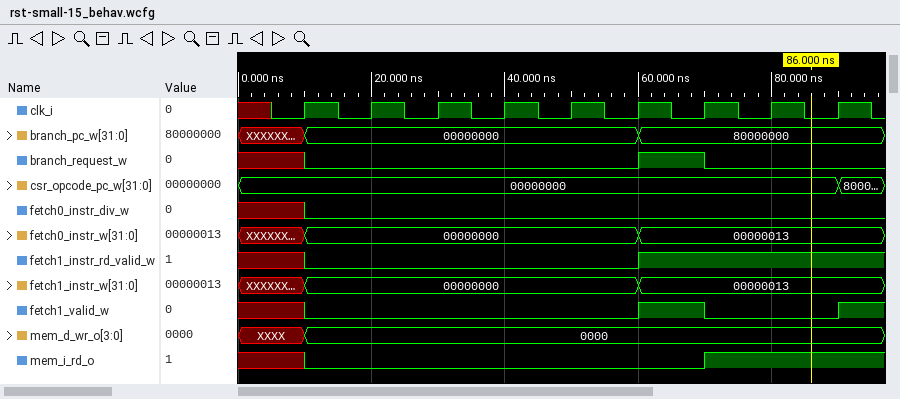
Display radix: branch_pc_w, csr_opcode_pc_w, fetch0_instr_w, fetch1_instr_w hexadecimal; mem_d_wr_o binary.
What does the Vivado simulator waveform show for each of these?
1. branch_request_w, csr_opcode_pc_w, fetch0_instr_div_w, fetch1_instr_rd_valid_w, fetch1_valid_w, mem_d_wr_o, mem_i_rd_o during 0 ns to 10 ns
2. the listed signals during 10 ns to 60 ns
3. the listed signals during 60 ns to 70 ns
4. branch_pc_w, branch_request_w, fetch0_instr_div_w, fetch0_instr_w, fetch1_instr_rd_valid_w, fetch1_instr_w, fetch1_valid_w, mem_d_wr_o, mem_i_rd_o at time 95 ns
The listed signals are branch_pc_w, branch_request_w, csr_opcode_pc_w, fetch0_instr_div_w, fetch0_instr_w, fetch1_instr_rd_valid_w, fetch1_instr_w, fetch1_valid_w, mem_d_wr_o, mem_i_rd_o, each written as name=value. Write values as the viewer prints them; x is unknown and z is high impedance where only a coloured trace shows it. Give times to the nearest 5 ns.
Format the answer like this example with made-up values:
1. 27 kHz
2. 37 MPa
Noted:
1. branch_request_w=x, csr_opcode_pc_w=00000000, fetch0_instr_div_w=x, fetch1_instr_rd_valid_w=x, fetch1_valid_w=x, mem_d_wr_o=XXXX, mem_i_rd_o=x
2. branch_pc_w=00000000, branch_request_w=0, csr_opcode_pc_w=00000000, fetch0_instr_div_w=0, fetch0_instr_w=00000000, fetch1_instr_rd_valid_w=0, fetch1_instr_w=00000000, fetch1_valid_w=0, mem_d_wr_o=0000, mem_i_rd_o=0
3. branch_pc_w=80000000, branch_request_w=1, csr_opcode_pc_w=00000000, fetch0_instr_div_w=0, fetch0_instr_w=00000013, fetch1_instr_rd_valid_w=1, fetch1_instr_w=00000013, fetch1_valid_w=1, mem_d_wr_o=0000, mem_i_rd_o=0
4. branch_pc_w=80000000, branch_request_w=0, fetch0_instr_div_w=0, fetch0_instr_w=00000013, fetch1_instr_rd_valid_w=1, fetch1_instr_w=00000013, fetch1_valid_w=1, mem_d_wr_o=0000, mem_i_rd_o=1
